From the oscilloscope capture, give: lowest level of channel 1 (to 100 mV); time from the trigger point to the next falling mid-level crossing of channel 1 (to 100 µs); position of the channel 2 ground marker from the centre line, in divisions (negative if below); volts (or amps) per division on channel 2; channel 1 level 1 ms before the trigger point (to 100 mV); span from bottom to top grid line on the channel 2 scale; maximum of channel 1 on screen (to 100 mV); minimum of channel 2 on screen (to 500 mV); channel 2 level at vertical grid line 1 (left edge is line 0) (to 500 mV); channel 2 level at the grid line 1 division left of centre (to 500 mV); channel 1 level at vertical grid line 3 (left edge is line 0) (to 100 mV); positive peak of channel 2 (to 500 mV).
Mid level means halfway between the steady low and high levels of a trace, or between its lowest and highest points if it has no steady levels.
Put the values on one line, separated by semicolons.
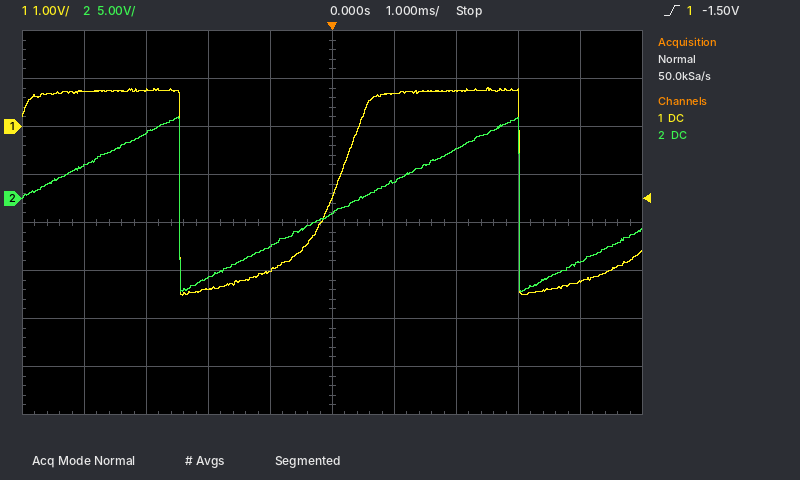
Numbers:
-3.5 V; 3.0 ms; +0.5 div; 5 V; -3.0 V; 40 V; 800 mV; -9.5 V; 3.5 V; -5.0 V; -3.4 V; 8.5 V
